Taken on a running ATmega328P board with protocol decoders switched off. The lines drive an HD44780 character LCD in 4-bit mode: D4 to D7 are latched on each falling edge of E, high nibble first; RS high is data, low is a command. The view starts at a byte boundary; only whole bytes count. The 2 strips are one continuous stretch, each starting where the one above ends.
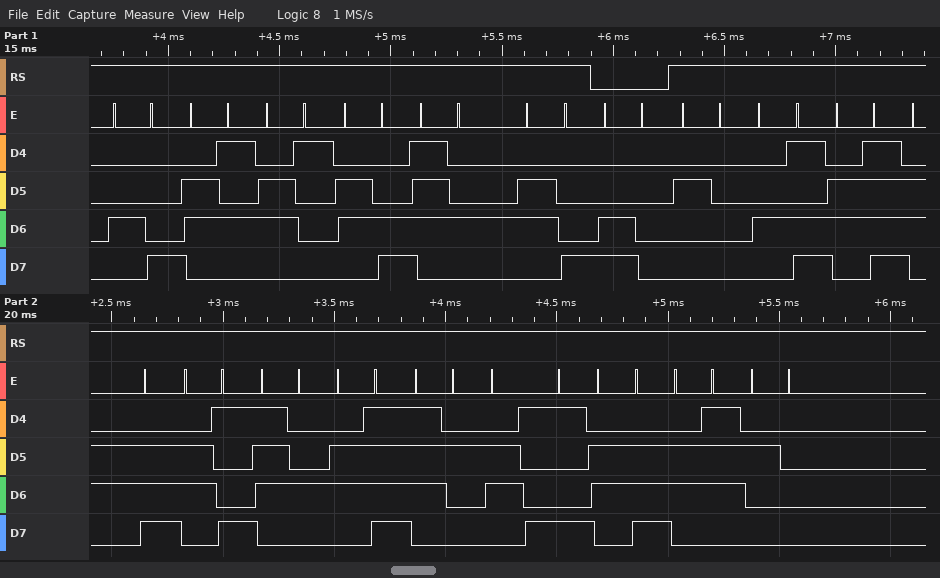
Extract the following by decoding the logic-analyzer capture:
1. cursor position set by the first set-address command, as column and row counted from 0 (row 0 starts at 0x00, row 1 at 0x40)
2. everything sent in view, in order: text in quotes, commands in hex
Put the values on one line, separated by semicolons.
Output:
column 0, row 1; "Health" 0xC0 " Monitoring "
